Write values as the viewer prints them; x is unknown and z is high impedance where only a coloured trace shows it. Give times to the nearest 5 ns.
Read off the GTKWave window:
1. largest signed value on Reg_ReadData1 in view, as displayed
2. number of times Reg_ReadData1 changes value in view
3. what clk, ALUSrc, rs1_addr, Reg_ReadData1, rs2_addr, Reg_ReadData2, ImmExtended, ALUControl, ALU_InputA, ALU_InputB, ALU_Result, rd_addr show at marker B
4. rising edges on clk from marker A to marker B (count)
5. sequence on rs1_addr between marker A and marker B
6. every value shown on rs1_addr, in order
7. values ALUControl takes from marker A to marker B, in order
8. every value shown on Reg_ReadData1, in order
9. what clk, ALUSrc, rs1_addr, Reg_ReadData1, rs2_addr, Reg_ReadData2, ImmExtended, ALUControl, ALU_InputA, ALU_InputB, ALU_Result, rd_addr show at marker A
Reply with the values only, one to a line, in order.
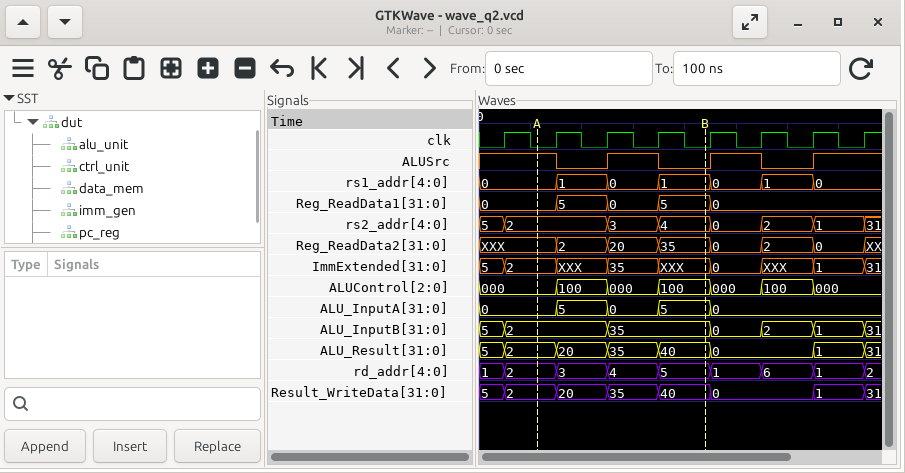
5
4
clk=0, ALUSrc=0, rs1_addr=1, Reg_ReadData1=5, rs2_addr=4, Reg_ReadData2=35, ImmExtended=XXX, ALUControl=100, ALU_InputA=5, ALU_InputB=35, ALU_Result=40, rd_addr=5
3
0, 1, 0, 1
0, 1, 0, 1, 0, 1, 0
000, 100, 000, 100
0, 5, 0, 5, 0
clk=0, ALUSrc=1, rs1_addr=0, Reg_ReadData1=0, rs2_addr=2, Reg_ReadData2=XXX, ImmExtended=2, ALUControl=000, ALU_InputA=0, ALU_InputB=2, ALU_Result=2, rd_addr=2
